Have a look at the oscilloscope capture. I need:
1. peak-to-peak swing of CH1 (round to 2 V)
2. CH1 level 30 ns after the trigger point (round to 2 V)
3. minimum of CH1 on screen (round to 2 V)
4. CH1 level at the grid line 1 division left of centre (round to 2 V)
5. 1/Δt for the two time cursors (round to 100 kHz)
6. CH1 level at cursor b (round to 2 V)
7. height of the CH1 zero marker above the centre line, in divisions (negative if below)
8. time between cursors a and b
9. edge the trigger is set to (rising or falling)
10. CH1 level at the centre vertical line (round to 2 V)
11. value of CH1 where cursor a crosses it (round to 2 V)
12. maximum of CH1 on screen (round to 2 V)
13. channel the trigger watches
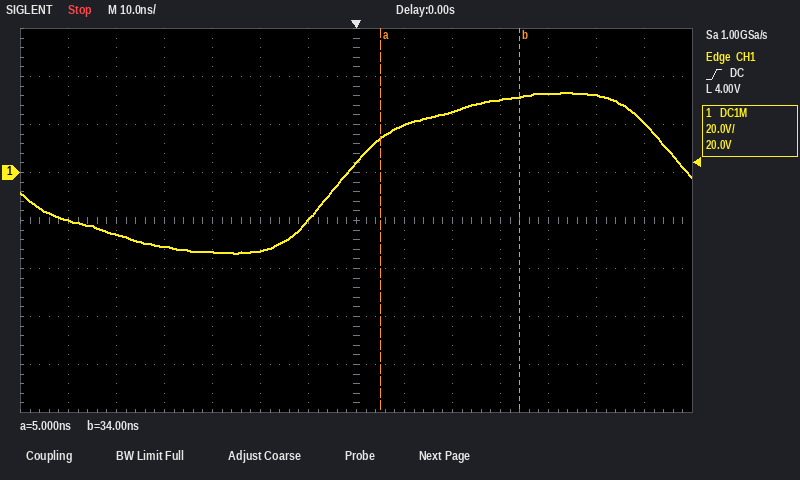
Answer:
68 V
30 V
-34 V
-20 V
34.5 MHz
32 V
+1.0 div
29 ns
rising
4 V
14 V
34 V
CH1
